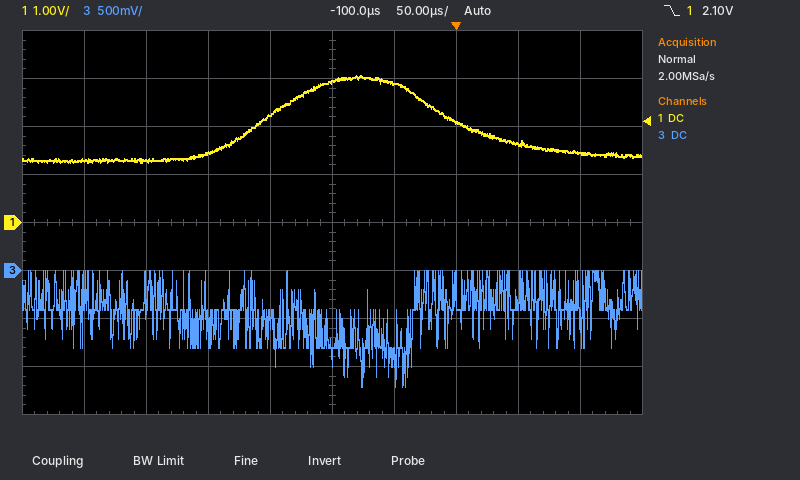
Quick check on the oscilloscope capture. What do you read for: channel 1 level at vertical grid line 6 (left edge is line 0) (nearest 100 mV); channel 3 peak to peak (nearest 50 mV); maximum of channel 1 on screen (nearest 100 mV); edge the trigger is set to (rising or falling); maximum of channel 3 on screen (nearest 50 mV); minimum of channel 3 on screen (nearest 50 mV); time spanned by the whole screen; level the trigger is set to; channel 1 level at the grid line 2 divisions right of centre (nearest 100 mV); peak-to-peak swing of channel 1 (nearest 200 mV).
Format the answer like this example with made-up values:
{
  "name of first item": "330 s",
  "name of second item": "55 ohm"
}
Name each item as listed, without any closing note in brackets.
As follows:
{
  "channel 1 level at vertical grid line 6 (left edge is line 0)": "2.9 V",
  "channel 3 peak to peak": "1.20 V",
  "maximum of channel 1 on screen": "3.1 V",
  "edge the trigger is set to": "falling",
  "maximum of channel 3 on screen": "0 mV",
  "minimum of channel 3 on screen": "-1.20 V",
  "time spanned by the whole screen": "500 µs",
  "level the trigger is set to": "2.10 V",
  "channel 1 level at the grid line 2 divisions right of centre": "2.1 V",
  "peak-to-peak swing of channel 1": "1.8 V"
}
